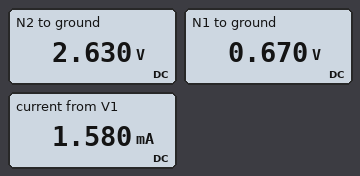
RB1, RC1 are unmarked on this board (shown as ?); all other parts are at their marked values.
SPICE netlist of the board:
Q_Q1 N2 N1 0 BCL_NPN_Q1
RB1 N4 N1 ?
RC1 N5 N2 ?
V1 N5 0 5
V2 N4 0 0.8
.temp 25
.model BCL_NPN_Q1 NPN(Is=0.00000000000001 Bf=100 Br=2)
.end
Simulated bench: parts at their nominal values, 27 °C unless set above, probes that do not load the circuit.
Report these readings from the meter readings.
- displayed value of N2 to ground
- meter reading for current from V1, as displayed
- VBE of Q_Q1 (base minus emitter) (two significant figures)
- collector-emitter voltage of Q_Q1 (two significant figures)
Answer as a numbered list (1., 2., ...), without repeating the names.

1. 2.630 V
2. 1.580 mA
3. 670 mV
4. 2.6 V
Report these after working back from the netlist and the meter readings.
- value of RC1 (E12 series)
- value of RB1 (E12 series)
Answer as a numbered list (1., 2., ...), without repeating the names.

1. 1.5 kΩ
2. 8.2 kΩ
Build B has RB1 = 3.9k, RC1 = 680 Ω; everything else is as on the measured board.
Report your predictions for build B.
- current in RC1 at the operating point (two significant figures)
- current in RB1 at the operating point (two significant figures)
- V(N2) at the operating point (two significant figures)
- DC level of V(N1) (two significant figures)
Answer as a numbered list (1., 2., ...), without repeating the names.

1. 2.9 mA
2. 29 µA
3. 3.0 V
4. 690 mV
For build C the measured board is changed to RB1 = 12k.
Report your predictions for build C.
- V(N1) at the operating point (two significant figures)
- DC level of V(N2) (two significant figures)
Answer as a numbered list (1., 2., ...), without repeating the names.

1. 660 mV
2. 3.3 V
